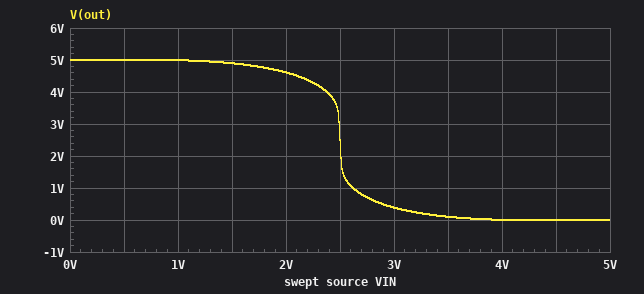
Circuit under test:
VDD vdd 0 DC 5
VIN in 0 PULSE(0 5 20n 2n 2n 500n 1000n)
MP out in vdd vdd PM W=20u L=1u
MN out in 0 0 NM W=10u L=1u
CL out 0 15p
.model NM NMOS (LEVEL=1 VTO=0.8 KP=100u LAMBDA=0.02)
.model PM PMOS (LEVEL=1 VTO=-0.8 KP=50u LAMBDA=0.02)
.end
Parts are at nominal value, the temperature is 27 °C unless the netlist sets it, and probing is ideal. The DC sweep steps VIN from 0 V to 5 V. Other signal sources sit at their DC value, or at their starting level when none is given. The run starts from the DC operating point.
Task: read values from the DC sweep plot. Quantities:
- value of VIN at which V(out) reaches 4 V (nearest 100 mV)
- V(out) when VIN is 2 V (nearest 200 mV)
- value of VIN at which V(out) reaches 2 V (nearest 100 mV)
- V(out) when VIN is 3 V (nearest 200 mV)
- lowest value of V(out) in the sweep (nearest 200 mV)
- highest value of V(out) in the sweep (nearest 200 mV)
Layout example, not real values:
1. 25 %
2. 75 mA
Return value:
1. 2.4 V
2. 4.6 V
3. 2.5 V
4. 400 mV
5. 0 V
6. 5.0 V
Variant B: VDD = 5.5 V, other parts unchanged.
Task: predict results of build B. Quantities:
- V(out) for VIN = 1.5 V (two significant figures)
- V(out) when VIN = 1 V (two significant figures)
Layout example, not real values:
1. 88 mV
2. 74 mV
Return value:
1. 5.4 V
2. 5.5 V
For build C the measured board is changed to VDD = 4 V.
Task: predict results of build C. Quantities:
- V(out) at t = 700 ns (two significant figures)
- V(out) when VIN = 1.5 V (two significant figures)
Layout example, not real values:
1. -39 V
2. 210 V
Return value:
1. 4.0 V
2. 3.8 V
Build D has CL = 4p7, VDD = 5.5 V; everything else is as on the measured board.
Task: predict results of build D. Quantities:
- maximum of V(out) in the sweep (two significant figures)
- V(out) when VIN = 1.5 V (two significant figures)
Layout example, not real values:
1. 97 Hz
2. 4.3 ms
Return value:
1. 5.5 V
2. 5.4 V
